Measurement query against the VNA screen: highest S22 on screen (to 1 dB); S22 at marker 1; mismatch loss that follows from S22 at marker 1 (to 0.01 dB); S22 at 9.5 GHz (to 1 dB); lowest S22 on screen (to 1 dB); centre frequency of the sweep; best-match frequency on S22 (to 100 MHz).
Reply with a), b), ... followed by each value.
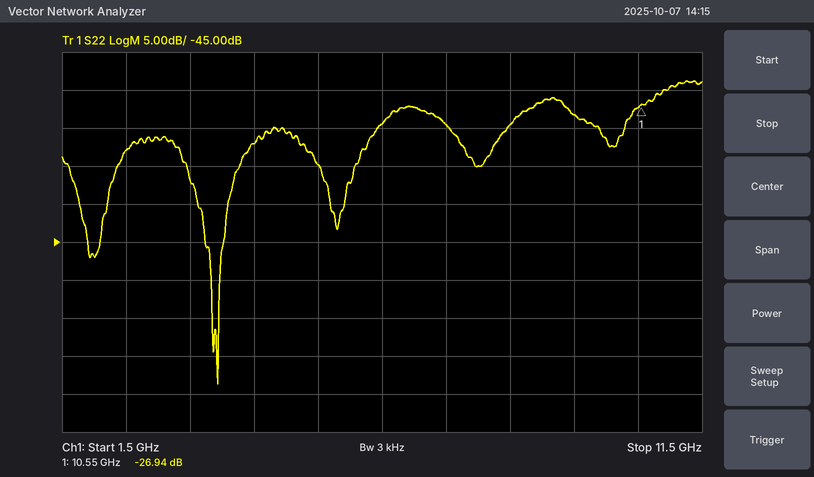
a) -24 dB
b) -26.94 dB
c) 0.01 dB
d) -28 dB
e) -64 dB
f) 6.5 GHz
g) 3.9 GHz
